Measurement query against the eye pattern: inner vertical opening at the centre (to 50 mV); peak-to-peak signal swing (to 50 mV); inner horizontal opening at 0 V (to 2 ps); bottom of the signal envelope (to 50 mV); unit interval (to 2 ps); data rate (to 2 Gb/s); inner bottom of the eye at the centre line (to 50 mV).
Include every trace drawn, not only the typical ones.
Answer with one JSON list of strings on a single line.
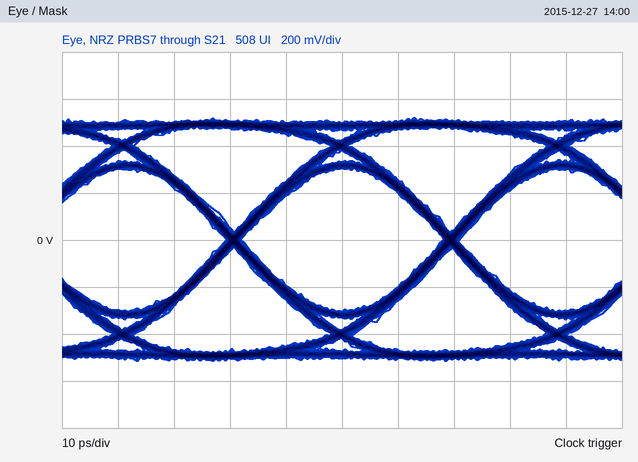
["600 mV", "1.05 V", "36 ps", "-500 mV", "38 ps", "26 Gb/s", "-300 mV"]
